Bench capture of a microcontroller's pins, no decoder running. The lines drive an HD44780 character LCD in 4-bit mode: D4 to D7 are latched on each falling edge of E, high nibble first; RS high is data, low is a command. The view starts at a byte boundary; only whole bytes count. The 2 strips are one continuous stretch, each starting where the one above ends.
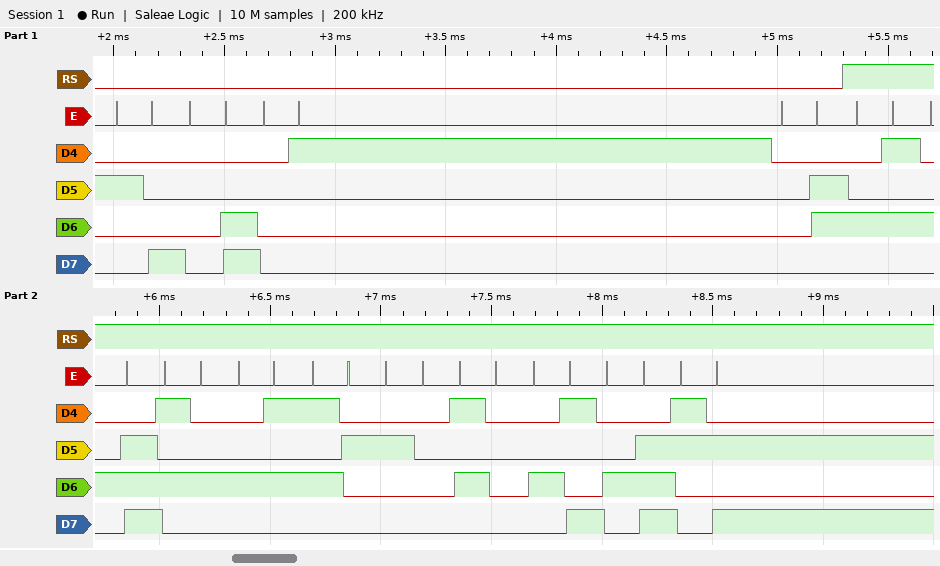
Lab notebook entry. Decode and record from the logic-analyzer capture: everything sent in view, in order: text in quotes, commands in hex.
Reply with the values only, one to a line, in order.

0x28 0x0C 0x01 0x06 "ENTER PIN:"
